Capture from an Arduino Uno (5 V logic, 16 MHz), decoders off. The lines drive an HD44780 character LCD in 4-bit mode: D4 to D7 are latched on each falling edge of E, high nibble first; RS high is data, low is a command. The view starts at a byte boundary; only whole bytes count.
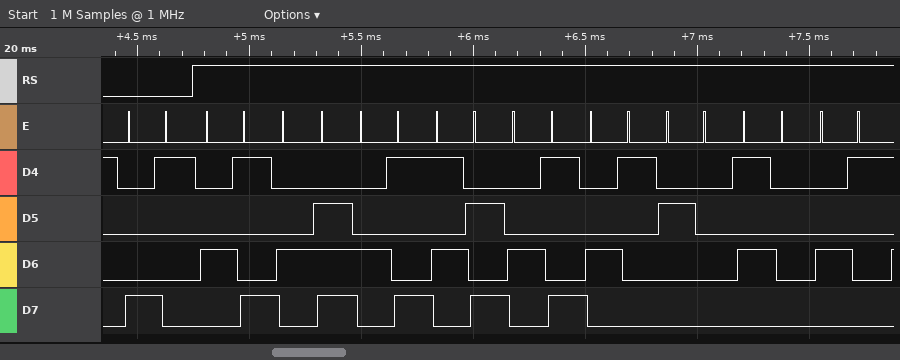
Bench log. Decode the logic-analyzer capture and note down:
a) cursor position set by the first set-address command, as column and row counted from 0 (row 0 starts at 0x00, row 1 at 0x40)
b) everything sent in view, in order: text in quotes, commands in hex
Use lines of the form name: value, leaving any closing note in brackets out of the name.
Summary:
cursor position set by the first set-address command, as column and row counted from 0: column 1, row 0
everything sent in view, in order: text in quotes, commands in hex: 0x81 "INIZIA PA"
